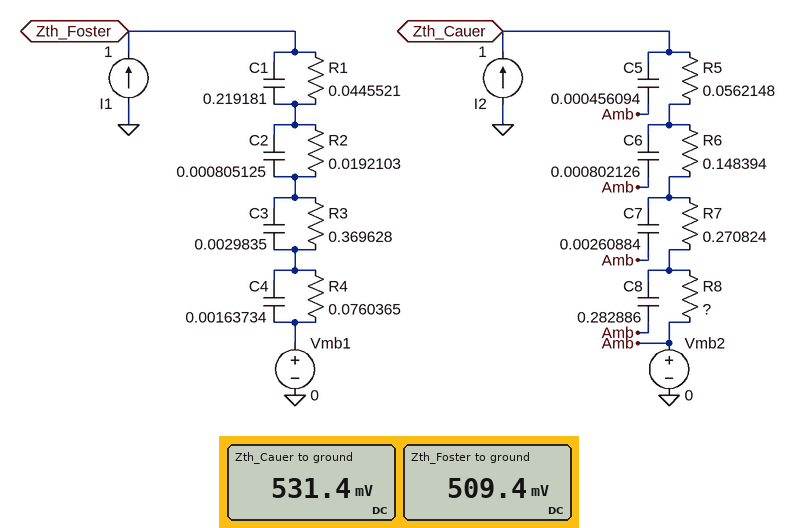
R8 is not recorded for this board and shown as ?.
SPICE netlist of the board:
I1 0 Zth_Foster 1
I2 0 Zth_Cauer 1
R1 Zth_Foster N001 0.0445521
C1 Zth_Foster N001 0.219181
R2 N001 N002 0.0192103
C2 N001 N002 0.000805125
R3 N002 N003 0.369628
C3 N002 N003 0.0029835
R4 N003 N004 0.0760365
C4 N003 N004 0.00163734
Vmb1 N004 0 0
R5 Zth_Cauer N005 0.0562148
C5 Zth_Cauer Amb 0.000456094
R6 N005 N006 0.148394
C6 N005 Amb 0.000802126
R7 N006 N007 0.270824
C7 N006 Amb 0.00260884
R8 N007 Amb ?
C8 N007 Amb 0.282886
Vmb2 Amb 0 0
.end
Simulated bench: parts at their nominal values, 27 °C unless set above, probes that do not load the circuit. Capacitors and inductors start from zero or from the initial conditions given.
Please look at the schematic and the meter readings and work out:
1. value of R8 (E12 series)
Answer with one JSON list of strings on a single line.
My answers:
["0.056 Ω"]
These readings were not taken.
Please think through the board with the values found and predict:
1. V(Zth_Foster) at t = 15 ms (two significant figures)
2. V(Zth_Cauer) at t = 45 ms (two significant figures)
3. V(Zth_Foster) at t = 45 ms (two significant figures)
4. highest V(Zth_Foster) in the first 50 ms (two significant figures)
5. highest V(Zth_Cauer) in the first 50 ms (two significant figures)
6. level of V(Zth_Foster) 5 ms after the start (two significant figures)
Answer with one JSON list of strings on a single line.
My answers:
["500 mV", "530 mV", "510 mV", "510 mV", "530 mV", "480 mV"]
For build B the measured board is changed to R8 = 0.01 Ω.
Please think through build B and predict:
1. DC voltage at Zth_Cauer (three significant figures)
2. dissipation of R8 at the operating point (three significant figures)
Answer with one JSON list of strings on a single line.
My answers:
["485 mV", "10.0 mW"]
